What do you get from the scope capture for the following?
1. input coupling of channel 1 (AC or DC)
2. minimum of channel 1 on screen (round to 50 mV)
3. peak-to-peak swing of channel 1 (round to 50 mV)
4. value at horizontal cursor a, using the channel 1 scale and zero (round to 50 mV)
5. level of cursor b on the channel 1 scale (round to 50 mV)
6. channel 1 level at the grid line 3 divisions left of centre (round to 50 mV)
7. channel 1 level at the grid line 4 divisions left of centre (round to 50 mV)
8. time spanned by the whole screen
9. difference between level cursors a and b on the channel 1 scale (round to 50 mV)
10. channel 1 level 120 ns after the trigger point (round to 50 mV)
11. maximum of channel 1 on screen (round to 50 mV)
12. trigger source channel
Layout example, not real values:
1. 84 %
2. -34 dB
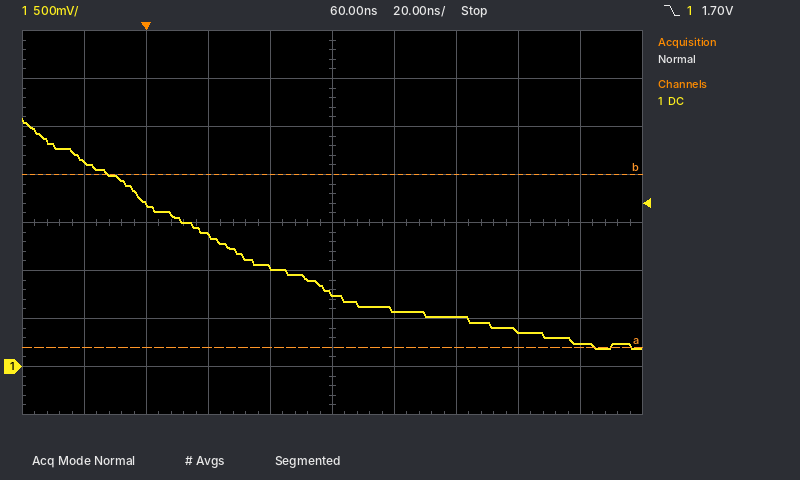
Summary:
1. DC
2. 200 mV
3. 2.40 V
4. 200 mV
5. 2.00 V
6. 1.70 V
7. 2.15 V
8. 200 ns
9. 1.80 V
10. 350 mV
11. 2.60 V
12. channel 1
